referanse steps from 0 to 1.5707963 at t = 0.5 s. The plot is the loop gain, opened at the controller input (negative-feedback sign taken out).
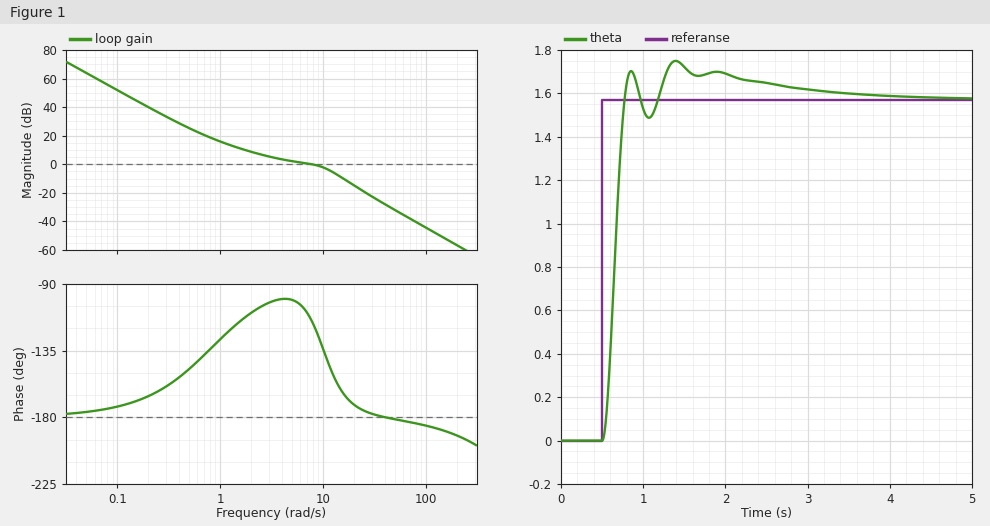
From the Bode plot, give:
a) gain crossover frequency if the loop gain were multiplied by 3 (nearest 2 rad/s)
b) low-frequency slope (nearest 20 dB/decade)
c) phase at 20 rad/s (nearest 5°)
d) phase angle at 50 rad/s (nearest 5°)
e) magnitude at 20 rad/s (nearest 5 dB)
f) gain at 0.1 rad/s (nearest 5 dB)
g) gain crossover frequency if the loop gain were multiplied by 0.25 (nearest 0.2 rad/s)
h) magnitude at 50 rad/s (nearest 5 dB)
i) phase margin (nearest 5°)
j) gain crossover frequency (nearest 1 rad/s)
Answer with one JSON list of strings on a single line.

["16 rad/s", "-40 dB/decade", "-170°", "-180°", "-15 dB", "50 dB", "1.4 rad/s", "-30 dB", "65°", "8 rad/s"]
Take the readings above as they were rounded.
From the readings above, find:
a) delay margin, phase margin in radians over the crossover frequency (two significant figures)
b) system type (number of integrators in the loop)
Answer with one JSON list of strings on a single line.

["0.14 s", "2"]
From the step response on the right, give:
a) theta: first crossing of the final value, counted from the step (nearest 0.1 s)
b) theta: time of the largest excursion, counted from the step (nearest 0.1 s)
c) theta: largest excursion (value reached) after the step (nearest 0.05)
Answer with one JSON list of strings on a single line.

["0.3 s", "0.9 s", "1.75"]
